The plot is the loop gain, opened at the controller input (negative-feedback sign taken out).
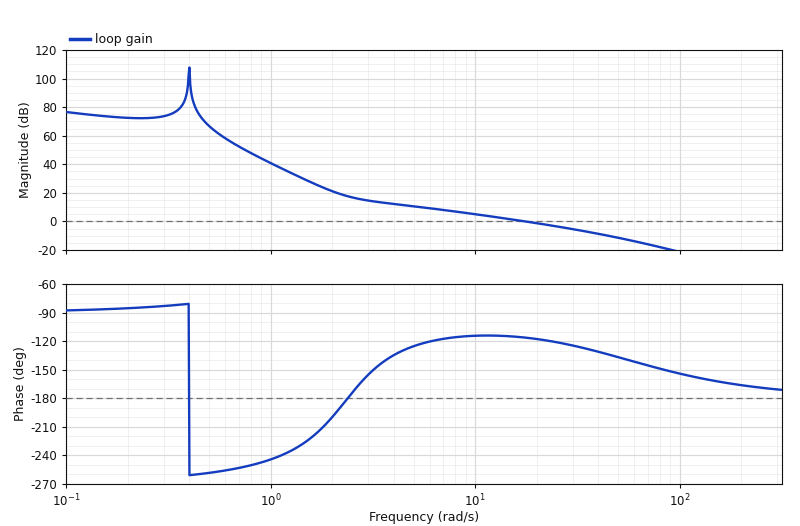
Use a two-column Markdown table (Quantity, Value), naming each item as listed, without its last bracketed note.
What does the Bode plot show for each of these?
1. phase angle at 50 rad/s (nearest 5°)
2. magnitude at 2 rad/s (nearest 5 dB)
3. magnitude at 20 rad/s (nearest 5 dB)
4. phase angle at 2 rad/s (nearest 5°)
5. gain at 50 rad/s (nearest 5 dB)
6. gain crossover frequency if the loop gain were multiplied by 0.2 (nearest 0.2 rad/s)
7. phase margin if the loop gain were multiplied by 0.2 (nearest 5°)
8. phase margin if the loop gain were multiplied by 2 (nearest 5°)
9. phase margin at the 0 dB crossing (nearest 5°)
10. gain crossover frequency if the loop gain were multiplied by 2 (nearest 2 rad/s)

| Quantity | Value |
|---|---|
| phase angle at 50 rad/s | -135° |
| magnitude at 2 rad/s | 20 dB |
| magnitude at 20 rad/s | 0 dB |
| phase angle at 2 rad/s | -200° |
| gain at 50 rad/s | -10 dB |
| gain crossover frequency if the loop gain were multiplied by 0.2 | 3.2 rad/s |
| phase margin if the loop gain were multiplied by 0.2 | 30° |
| phase margin if the loop gain were multiplied by 2 | 55° |
| phase margin at the 0 dB crossing | 65° |
| gain crossover frequency if the loop gain were multiplied by 2 | 32 rad/s |
